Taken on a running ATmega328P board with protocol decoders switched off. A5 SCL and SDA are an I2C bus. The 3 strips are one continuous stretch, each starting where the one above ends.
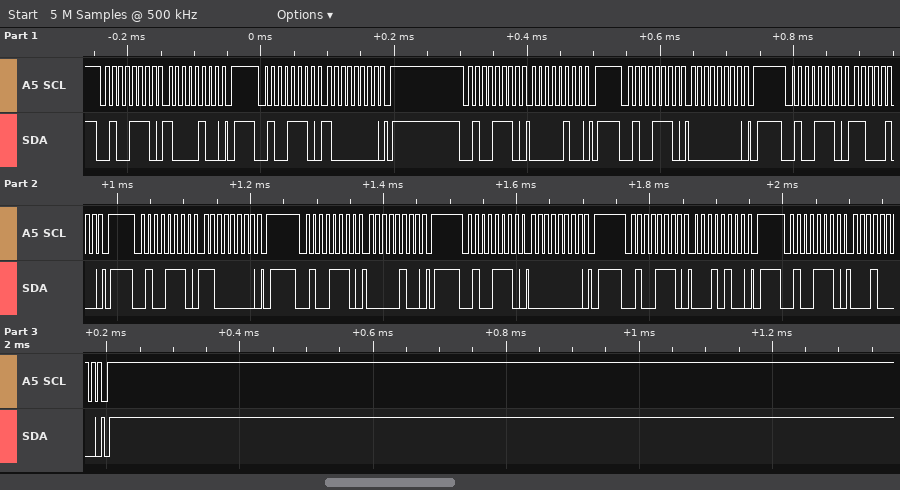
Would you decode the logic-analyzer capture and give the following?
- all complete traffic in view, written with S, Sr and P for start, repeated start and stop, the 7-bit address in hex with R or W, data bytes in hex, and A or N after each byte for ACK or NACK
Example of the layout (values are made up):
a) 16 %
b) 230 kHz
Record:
a) S 27W A 84 A P S 27W A 80 A P S 27W A 04 A P S 27W A 00 A P S 27W A C4 A P S 27W A C0 A P S 27W A 04 A P S 27W A 00 A P S 27W A 14 A P S 27W A 10 A P
